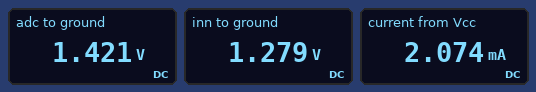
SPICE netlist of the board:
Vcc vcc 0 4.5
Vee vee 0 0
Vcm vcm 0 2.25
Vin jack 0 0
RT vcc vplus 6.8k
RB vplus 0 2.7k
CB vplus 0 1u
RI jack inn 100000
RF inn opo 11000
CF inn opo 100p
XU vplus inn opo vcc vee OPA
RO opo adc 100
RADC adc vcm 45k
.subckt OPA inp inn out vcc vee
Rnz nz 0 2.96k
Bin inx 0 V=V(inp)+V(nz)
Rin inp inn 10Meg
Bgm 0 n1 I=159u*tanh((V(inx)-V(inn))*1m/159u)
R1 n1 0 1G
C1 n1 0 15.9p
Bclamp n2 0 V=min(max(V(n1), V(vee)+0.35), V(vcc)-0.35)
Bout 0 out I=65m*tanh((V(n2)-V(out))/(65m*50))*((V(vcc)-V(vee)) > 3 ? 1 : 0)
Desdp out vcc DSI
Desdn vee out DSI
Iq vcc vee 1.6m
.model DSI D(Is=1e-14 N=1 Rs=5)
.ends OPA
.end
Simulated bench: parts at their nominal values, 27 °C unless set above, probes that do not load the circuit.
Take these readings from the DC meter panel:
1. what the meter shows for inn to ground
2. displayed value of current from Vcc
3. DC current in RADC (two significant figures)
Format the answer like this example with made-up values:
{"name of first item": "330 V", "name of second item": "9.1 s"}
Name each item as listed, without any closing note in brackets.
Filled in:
{"what the meter shows for inn to ground": "1.279 V", "displayed value of current from Vcc": "2.074 mA", "DC current in RADC": "18 µA"}
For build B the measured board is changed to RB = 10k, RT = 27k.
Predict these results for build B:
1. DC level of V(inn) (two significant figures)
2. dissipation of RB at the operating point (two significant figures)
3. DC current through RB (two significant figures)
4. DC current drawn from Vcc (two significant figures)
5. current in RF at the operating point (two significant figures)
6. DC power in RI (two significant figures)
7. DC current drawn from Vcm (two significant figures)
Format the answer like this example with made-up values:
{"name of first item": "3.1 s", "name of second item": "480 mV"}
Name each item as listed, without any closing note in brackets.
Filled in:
{"DC level of V(inn)": "1.2 V", "dissipation of RB at the operating point": "150 µW", "DC current through RB": "120 µA", "DC current drawn from Vcc": "1.7 mA", "current in RF at the operating point": "12 µA", "DC power in RI": "15 µW", "DC current drawn from Vcm": "20 µA"}
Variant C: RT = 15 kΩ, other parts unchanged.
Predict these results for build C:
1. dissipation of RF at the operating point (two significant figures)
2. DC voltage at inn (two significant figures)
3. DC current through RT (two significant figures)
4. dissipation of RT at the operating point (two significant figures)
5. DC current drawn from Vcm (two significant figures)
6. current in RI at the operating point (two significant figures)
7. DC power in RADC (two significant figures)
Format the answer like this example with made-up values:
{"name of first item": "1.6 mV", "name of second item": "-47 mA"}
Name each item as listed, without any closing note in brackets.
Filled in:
{"dissipation of RF at the operating point": "520 nW", "DC voltage at inn": "690 mV", "DC current through RT": "250 µA", "dissipation of RT at the operating point": "970 µW", "DC current drawn from Vcm": "33 µA", "current in RI at the operating point": "6.9 µA", "DC power in RADC": "49 µW"}
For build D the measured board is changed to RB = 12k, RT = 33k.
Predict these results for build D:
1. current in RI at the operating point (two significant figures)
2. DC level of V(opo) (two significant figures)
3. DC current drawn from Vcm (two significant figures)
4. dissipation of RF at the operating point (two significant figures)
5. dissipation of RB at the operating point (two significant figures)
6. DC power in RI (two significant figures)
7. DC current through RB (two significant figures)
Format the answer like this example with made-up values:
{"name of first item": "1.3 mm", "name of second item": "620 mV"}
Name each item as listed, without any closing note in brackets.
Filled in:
{"current in RI at the operating point": "12 µA", "DC level of V(opo)": "1.3 V", "DC current drawn from Vcm": "20 µA", "dissipation of RF at the operating point": "1.6 µW", "dissipation of RB at the operating point": "120 µW", "DC power in RI": "14 µW", "DC current through RB": "100 µA"}
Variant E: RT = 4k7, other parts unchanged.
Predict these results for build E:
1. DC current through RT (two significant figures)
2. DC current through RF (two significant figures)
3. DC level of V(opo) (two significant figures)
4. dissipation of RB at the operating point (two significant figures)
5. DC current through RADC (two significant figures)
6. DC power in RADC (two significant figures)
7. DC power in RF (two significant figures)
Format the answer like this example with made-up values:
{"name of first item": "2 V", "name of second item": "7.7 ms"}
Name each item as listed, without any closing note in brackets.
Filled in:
{"DC current through RT": "610 µA", "DC current through RF": "16 µA", "DC level of V(opo)": "1.8 V", "dissipation of RB at the operating point": "1.0 mW", "DC current through RADC": "9.5 µA", "DC power in RADC": "4.0 µW", "DC power in RF": "3.0 µW"}
